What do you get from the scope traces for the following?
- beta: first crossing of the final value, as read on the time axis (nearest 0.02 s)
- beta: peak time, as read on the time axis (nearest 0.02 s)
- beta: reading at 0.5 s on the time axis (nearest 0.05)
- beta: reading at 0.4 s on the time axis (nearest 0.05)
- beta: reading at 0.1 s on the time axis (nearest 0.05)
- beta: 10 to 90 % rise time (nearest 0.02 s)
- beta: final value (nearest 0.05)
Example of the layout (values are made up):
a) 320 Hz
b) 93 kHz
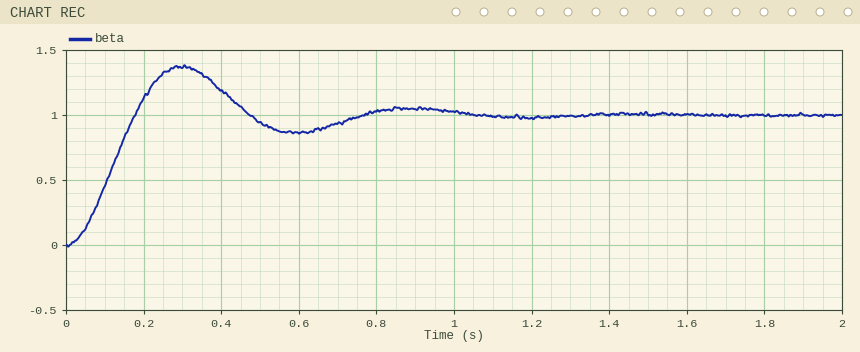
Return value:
a) 0.18 s
b) 0.30 s
c) 0.95
d) 1.20
e) 0.45
f) 0.12 s
g) 1.00
